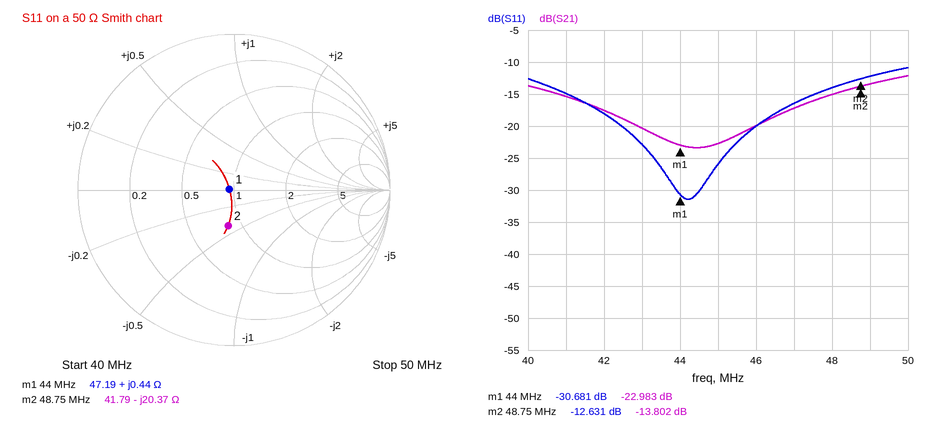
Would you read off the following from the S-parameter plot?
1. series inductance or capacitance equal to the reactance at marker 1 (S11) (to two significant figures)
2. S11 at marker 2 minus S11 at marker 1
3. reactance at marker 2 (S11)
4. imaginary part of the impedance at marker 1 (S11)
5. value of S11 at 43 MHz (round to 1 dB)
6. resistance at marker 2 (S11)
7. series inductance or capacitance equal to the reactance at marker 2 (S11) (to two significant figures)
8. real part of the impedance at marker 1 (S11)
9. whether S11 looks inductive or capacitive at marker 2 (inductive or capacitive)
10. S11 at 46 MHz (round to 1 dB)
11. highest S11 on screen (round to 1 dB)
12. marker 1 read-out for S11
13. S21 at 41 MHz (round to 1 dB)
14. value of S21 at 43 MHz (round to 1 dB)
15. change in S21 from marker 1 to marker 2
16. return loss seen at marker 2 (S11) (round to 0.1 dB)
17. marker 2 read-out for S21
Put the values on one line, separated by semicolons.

1.6 nH; 18.050 dB; -20.37 Ω; +0.44 Ω; -23 dB; 41.79 Ω; 160 pF; 47.19 Ω; capacitive; -20 dB; -11 dB; -30.681 dB; -15 dB; -20 dB; 9.181 dB; 12.6 dB; -13.802 dB
